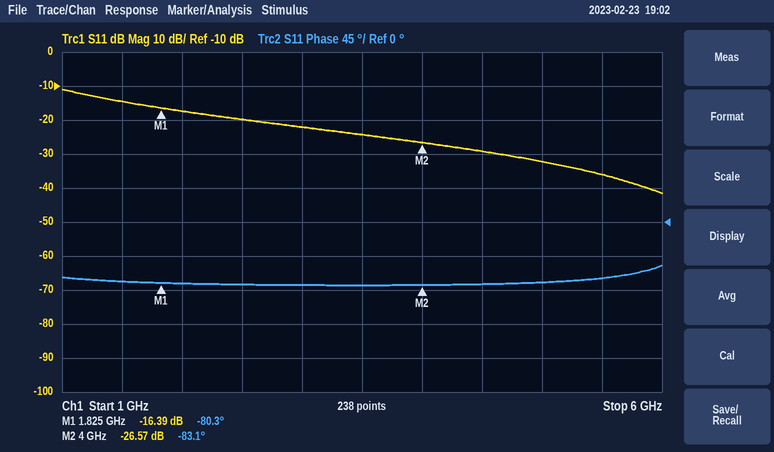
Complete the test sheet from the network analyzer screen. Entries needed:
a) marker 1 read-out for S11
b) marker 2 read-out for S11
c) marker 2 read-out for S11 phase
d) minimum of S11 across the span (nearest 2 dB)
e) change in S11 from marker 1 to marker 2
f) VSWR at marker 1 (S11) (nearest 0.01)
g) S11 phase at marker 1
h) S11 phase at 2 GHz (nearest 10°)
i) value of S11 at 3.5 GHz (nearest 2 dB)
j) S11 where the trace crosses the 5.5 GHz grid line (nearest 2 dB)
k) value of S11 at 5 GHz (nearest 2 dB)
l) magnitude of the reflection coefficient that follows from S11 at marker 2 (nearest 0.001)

-16.39 dB
-26.57 dB
-83.1°
-42 dB
-10.18 dB
1.36
-80.3°
-80°
-24 dB
-36 dB
-32 dB
0.047
